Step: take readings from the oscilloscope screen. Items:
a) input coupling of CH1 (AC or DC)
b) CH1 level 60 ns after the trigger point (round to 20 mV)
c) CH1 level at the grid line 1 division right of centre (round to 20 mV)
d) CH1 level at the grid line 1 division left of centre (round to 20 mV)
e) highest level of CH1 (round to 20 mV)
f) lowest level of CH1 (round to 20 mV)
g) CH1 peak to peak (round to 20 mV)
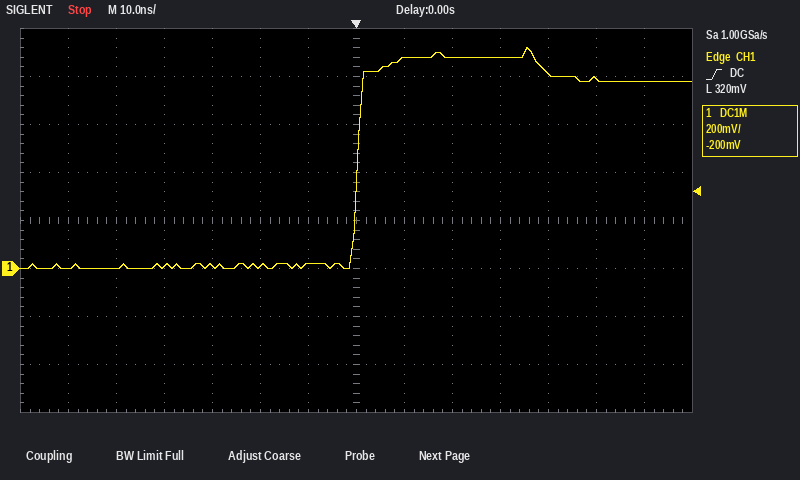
DC
780 mV
880 mV
20 mV
920 mV
0 mV
920 mV
